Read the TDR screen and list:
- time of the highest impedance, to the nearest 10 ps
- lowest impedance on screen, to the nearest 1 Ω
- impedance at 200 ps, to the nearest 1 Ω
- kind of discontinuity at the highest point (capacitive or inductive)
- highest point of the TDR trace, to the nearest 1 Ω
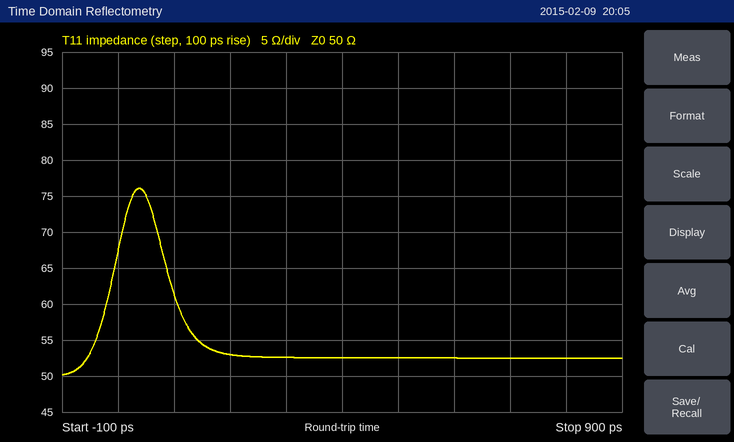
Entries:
40 ps
50 Ω
53 Ω
inductive
76 Ω
